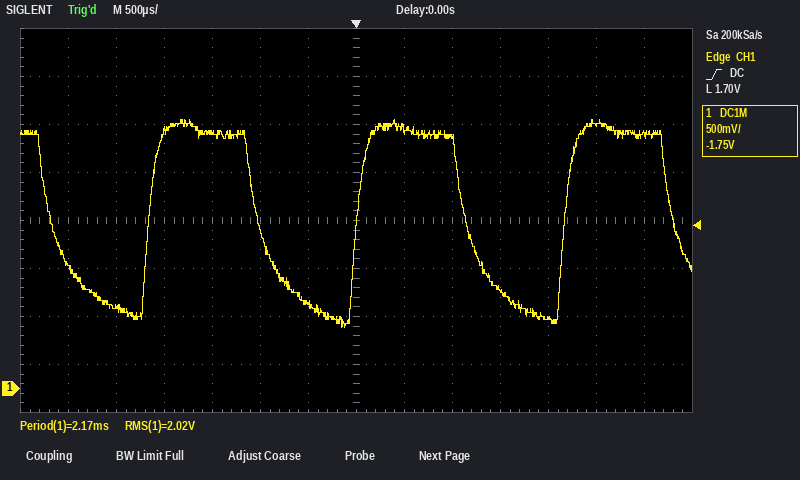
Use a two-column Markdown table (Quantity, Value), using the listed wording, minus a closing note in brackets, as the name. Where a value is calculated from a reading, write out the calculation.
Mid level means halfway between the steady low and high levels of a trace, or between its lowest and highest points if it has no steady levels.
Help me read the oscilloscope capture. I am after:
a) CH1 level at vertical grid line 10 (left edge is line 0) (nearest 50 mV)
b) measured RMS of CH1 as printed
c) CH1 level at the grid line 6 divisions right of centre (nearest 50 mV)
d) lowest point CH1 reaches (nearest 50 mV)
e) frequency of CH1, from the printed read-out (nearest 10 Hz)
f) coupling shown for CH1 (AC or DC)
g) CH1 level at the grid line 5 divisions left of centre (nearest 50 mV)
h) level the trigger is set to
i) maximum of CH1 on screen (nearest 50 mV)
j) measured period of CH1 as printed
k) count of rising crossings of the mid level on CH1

| Quantity | Value |
|---|---|
| CH1 level at vertical grid line 10 (left edge is line 0) | 1.05 V |
| measured RMS of CH1 as printed | 2.02 V |
| CH1 level at the grid line 6 divisions right of centre | 2.65 V |
| lowest point CH1 reaches | 650 mV |
| frequency of CH1, from the printed read-out | 1 / 2.17 ms ≈ 461 Hz, so 460 Hz to the nearest 10 Hz |
| coupling shown for CH1 | DC |
| CH1 level at the grid line 5 divisions left of centre | 850 mV |
| level the trigger is set to | 1.70 V |
| maximum of CH1 on screen | 2.80 V |
| measured period of CH1 as printed | 2.17 ms |
| count of rising crossings of the mid level on CH1 | 3 |
